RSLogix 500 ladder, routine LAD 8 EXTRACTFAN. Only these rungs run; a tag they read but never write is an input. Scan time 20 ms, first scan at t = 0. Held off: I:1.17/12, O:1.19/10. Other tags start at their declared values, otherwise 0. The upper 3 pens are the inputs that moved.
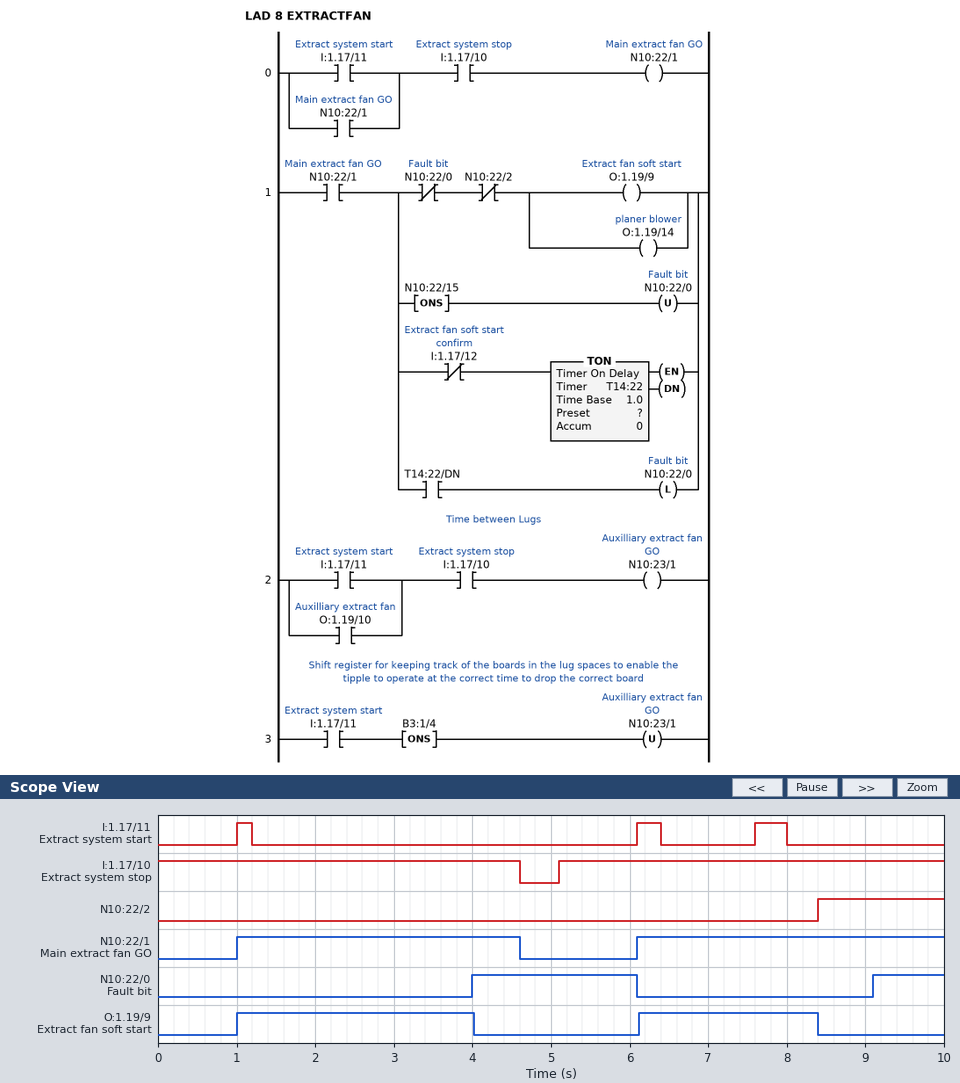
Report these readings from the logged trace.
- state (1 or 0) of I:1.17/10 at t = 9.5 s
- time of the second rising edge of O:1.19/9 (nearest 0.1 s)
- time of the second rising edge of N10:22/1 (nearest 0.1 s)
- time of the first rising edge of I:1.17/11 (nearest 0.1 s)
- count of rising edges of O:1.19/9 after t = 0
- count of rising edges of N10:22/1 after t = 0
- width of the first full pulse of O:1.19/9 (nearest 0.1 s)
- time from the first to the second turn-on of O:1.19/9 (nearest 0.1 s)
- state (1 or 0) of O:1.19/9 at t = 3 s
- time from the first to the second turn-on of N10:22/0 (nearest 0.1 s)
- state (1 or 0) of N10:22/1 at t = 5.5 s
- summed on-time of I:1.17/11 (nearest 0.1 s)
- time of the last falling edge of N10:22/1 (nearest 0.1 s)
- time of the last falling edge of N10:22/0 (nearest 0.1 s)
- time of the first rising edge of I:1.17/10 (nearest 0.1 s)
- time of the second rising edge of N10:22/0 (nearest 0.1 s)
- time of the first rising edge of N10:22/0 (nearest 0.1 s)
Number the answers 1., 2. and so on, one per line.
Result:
1. 1
2. 6.1 s
3. 6.1 s
4. 1.0 s
5. 2
6. 2
7. 3.0 s
8. 5.1 s
9. 1
10. 5.1 s
11. 0
12. 0.9 s
13. 4.6 s
14. 6.1 s
15. 5.1 s
16. 9.1 s
17. 4.0 s
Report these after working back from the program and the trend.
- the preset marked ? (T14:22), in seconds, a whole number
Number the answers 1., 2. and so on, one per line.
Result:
1. 3 s
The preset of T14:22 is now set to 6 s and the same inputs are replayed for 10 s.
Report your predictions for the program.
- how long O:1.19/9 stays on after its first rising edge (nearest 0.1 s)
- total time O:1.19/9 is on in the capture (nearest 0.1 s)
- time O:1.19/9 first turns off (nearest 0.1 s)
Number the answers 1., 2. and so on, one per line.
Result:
1. 3.6 s
2. 5.9 s
3. 4.6 s
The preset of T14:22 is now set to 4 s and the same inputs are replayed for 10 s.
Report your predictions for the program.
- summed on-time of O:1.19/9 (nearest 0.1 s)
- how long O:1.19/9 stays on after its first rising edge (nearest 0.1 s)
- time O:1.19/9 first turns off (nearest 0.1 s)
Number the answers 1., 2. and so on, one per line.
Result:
1. 5.9 s
2. 3.6 s
3. 4.6 s
